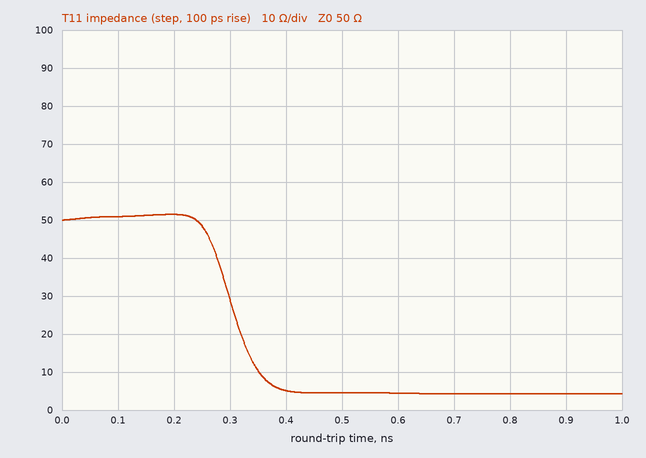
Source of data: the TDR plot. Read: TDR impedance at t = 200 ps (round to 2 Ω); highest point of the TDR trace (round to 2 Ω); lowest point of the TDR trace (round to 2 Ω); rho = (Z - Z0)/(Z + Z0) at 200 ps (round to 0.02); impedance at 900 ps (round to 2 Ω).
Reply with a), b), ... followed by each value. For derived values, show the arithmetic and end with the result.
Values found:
a) 52 Ω
b) 52 Ω
c) 4 Ω
d) (52 − 50)/(52 + 50) ≈ +0.02
e) 4 Ω
